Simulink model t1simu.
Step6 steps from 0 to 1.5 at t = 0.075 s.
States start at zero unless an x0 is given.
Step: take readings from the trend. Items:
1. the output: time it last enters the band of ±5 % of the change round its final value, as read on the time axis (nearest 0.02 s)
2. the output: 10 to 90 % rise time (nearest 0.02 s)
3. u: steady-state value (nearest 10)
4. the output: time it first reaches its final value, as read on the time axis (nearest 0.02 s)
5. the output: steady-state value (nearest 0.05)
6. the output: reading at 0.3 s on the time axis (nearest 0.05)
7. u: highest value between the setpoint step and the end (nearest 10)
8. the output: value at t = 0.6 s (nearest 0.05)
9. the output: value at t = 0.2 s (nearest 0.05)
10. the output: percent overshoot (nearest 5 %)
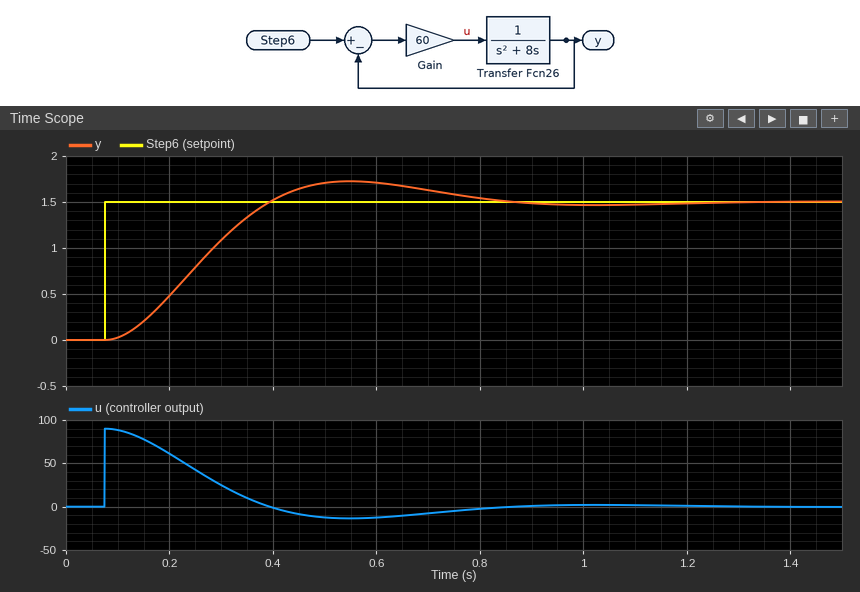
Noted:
0.76 s
0.22 s
0
0.40 s
1.50
1.10
90
1.70
0.50
15 %
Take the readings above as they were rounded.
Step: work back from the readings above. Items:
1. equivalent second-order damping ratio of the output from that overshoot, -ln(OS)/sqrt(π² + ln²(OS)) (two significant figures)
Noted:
0.52
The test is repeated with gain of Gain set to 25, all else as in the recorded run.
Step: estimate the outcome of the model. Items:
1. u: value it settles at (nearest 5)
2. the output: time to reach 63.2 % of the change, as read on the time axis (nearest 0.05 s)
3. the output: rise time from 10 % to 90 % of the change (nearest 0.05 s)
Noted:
0
0.45 s
0.50 s
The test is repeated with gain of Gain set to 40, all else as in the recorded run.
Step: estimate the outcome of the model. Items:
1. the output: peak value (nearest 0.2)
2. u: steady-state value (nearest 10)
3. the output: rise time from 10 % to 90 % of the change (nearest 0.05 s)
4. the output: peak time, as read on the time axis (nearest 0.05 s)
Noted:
1.6
0
0.30 s
0.70 s
